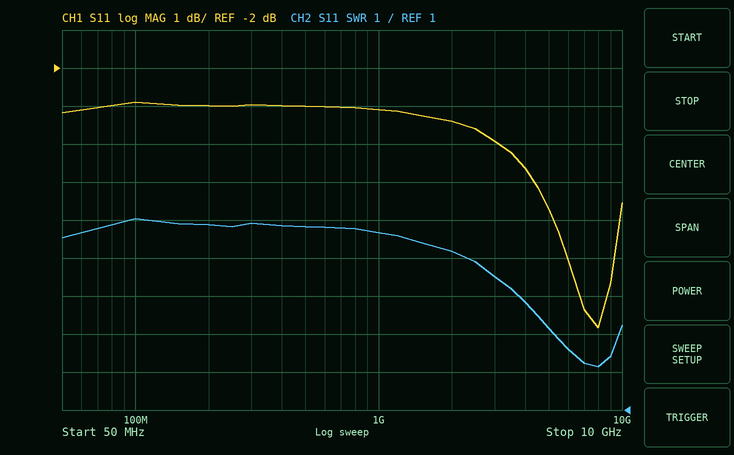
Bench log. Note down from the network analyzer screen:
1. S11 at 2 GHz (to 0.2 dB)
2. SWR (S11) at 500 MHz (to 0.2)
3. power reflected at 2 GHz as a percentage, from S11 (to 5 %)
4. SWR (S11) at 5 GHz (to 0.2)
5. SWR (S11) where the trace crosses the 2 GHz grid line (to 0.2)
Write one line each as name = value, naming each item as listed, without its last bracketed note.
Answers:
S11 at 2 GHz = -3.4 dB
SWR (S11) at 500 MHz = 5.8
power reflected at 2 GHz as a percentage, from S11 = 45 %
SWR (S11) at 5 GHz = 3.2
SWR (S11) where the trace crosses the 2 GHz grid line = 5.2
